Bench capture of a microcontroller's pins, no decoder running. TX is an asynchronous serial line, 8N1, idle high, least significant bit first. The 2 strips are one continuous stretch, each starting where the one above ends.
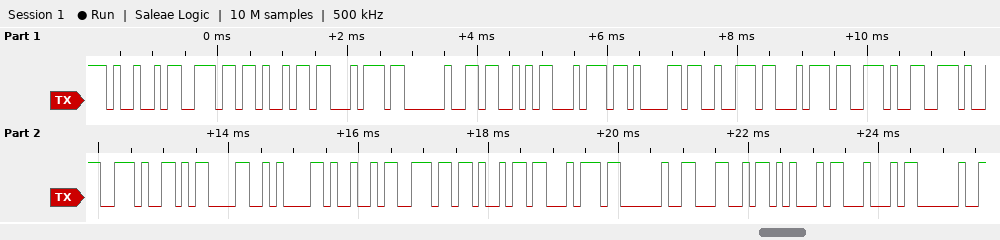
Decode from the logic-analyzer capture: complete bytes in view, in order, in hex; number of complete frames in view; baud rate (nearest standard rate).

49 6E 69 74 20 53 74 61 72 74 2E 2E 2E 0D 0A 49 6E 69 74 20 4C 45 44 20
24
9600 baud
